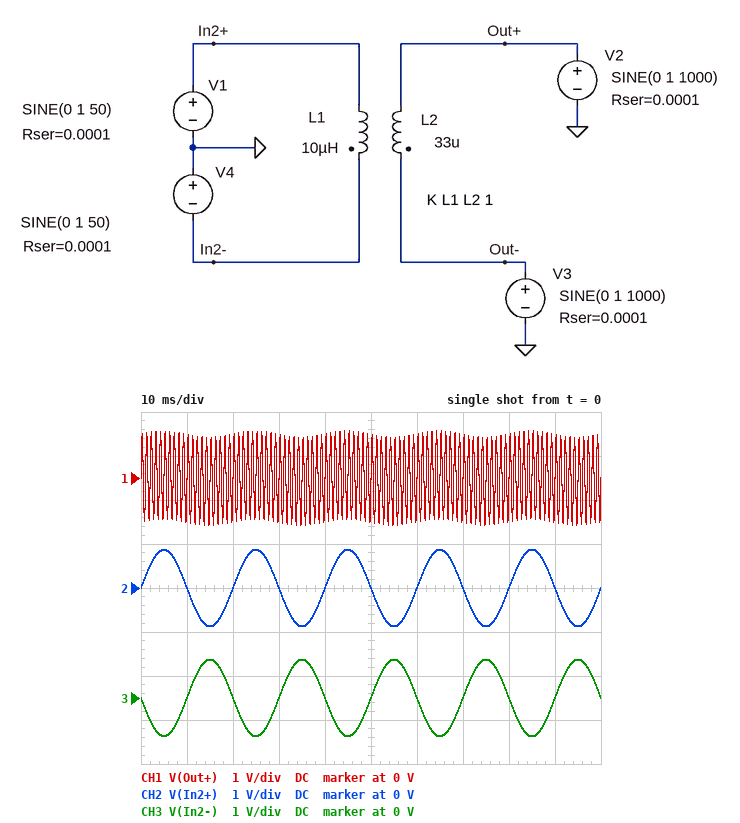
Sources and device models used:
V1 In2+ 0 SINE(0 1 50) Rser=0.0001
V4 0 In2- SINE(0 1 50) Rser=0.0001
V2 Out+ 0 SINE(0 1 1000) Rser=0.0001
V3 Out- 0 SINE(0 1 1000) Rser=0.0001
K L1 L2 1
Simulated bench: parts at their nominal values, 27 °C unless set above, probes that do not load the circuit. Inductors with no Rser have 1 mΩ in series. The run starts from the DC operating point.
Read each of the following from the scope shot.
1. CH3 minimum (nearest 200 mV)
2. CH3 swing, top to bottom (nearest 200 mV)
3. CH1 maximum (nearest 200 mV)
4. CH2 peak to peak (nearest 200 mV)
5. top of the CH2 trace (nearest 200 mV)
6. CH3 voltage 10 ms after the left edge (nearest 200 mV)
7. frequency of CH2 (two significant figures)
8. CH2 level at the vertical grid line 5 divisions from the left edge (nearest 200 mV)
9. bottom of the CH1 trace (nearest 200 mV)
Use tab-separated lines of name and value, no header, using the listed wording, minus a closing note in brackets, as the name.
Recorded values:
CH3 minimum	-800 mV
CH3 swing, top to bottom	1.8 V
CH1 maximum	1.0 V
CH2 peak to peak	1.8 V
top of the CH2 trace	800 mV
CH3 voltage 10 ms after the left edge	0 V
frequency of CH2	50 Hz
CH2 level at the vertical grid line 5 divisions from the left edge	0 V
bottom of the CH1 trace	-1.0 V
